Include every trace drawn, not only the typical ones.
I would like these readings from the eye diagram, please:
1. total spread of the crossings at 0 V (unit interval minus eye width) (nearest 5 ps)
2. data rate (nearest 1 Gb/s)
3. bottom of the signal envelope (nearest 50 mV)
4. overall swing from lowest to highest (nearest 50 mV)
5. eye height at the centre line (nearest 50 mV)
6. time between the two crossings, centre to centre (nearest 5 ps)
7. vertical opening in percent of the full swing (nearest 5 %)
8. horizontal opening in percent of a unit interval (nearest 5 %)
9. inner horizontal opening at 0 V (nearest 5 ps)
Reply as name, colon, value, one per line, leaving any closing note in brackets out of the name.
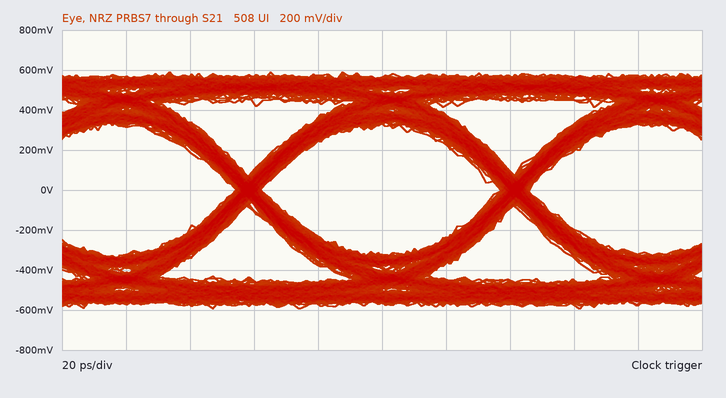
total spread of the crossings at 0 V (unit interval minus eye width): 10 ps
data rate: 12 Gb/s
bottom of the signal envelope: -600 mV
overall swing from lowest to highest: 1.20 V
eye height at the centre line: 650 mV
time between the two crossings, centre to centre: 85 ps
vertical opening in percent of the full swing: 55 %
horizontal opening in percent of a unit interval: 90 %
inner horizontal opening at 0 V: 75 ps
